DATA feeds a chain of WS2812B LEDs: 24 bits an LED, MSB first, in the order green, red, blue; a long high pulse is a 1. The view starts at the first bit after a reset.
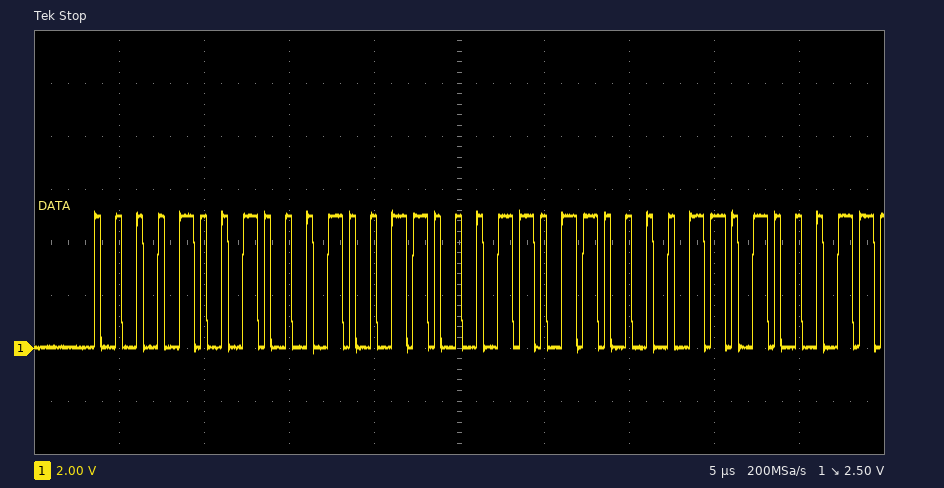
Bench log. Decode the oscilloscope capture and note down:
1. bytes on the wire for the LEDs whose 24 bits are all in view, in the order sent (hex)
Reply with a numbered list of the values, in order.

1. 09 13 1B
